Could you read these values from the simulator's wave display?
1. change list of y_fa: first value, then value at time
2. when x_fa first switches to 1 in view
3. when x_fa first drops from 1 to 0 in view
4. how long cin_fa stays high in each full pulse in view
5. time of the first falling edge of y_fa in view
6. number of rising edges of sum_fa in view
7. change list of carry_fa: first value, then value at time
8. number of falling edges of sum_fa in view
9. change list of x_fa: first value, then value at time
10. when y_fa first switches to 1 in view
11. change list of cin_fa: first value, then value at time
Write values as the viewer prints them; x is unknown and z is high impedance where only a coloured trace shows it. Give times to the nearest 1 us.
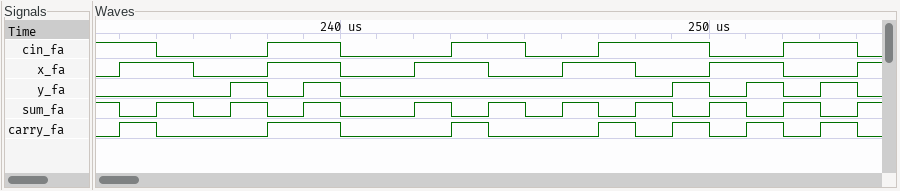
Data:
0, 1 at 237 us, 0 at 238 us, 1 at 239 us, 0 at 240 us, 1 at 249 us, 0 at 250 us, 1 at 251 us, 0 at 252 us, 1 at 253 us, 0 at 254 us
234 us
236 us
2 us, 2 us, 3 us, 2 us
238 us
10
0, 1 at 234 us, 0 at 235 us, 1 at 238 us, 0 at 240 us, 1 at 243 us, 0 at 244 us, 1 at 247 us, 0 at 248 us, 1 at 249 us, 0 at 250 us, 1 at 251 us, 0 at 252 us, 1 at 253 us, 0 at 254 us
10
0, 1 at 234 us, 0 at 236 us, 1 at 238 us, 0 at 240 us, 1 at 242 us, 0 at 244 us, 1 at 246 us, 0 at 248 us, 1 at 250 us, 0 at 252 us, 1 at 254 us
237 us
1, 0 at 235 us, 1 at 238 us, 0 at 240 us, 1 at 243 us, 0 at 245 us, 1 at 247 us, 0 at 250 us, 1 at 252 us, 0 at 254 us
